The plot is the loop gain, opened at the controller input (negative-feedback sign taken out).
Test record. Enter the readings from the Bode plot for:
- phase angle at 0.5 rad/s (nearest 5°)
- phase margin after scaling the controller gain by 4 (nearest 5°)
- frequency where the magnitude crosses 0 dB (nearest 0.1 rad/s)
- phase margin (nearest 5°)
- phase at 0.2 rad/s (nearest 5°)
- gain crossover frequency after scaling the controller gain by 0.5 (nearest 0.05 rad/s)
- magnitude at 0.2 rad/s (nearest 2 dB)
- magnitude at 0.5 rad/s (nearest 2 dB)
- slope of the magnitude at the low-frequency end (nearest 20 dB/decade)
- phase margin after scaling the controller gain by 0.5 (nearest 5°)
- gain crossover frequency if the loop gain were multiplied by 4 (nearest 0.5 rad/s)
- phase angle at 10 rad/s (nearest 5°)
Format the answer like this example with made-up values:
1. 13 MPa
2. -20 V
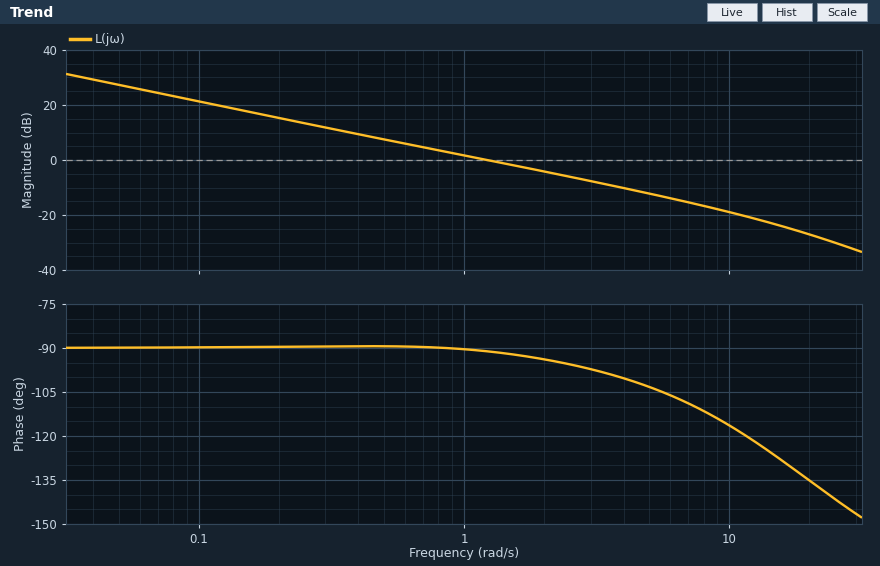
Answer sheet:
1. -90°
2. 75°
3. 1.2 rad/s
4. 90°
5. -90°
6. 0.60 rad/s
7. 16 dB
8. 8 dB
9. -20 dB/decade
10. 90°
11. 5.0 rad/s
12. -115°
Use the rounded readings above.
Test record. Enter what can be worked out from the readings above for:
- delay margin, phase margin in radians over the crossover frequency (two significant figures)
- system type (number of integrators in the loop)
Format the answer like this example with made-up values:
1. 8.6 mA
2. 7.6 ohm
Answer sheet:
1. 1.3 s
2. 1
